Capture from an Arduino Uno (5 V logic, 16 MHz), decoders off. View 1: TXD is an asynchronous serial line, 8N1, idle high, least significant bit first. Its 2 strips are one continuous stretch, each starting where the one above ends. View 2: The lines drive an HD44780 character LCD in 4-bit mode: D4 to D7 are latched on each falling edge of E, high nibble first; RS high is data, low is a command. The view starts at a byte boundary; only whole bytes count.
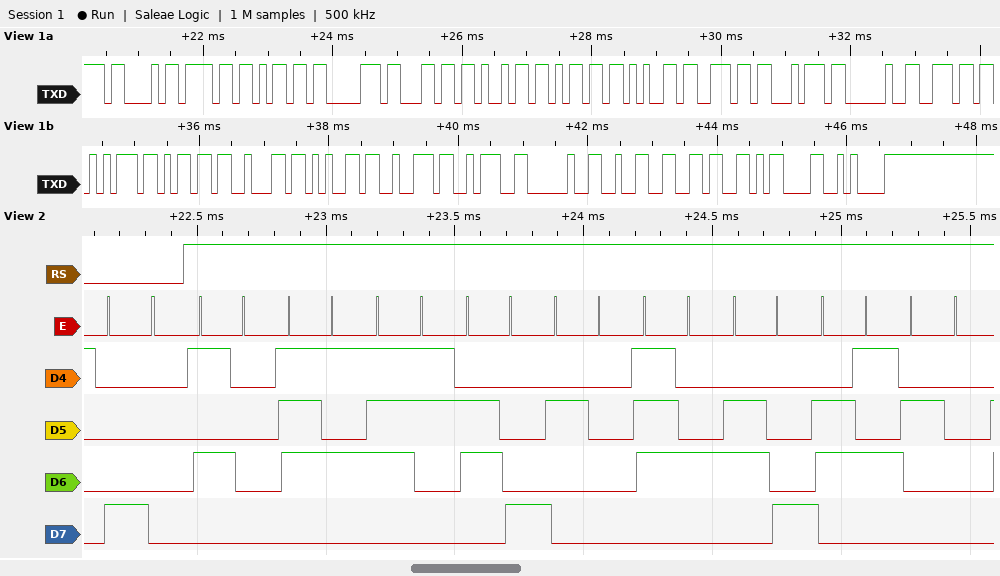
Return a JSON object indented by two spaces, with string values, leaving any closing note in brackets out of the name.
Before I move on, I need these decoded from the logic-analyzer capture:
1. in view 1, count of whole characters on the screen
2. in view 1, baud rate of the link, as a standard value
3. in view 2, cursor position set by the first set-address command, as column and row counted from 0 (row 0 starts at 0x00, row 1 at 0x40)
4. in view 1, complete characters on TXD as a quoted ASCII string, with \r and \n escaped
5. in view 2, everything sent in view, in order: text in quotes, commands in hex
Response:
{
  "in view 1, count of whole characters on the screen": "23",
  "in view 1, baud rate of the link, as a standard value": "9600 baud",
  "in view 2, cursor position set by the first set-address command, as column and row counted from 0": "column 0, row 0",
  "in view 1, complete characters on TXD as a quoted ASCII string, with \\r and \\n escaped": "\"Compliment number: 26\\r\\n\"",
  "in view 2, everything sent in view, in order: text in quotes, commands in hex": "0x80 \"Push the \""
}
